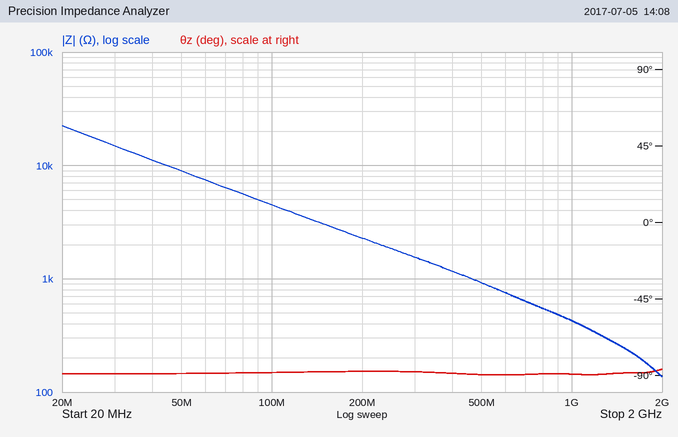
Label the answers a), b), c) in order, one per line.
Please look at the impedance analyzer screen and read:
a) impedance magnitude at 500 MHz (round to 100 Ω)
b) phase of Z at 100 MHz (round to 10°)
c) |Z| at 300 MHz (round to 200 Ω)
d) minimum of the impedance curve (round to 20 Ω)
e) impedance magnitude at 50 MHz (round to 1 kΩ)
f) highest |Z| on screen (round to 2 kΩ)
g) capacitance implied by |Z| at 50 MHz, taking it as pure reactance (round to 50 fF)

a) 900 Ω
b) -90°
c) 1.6 kΩ
d) 140 Ω
e) 9 kΩ
f) 22 kΩ
g) 350 fF
